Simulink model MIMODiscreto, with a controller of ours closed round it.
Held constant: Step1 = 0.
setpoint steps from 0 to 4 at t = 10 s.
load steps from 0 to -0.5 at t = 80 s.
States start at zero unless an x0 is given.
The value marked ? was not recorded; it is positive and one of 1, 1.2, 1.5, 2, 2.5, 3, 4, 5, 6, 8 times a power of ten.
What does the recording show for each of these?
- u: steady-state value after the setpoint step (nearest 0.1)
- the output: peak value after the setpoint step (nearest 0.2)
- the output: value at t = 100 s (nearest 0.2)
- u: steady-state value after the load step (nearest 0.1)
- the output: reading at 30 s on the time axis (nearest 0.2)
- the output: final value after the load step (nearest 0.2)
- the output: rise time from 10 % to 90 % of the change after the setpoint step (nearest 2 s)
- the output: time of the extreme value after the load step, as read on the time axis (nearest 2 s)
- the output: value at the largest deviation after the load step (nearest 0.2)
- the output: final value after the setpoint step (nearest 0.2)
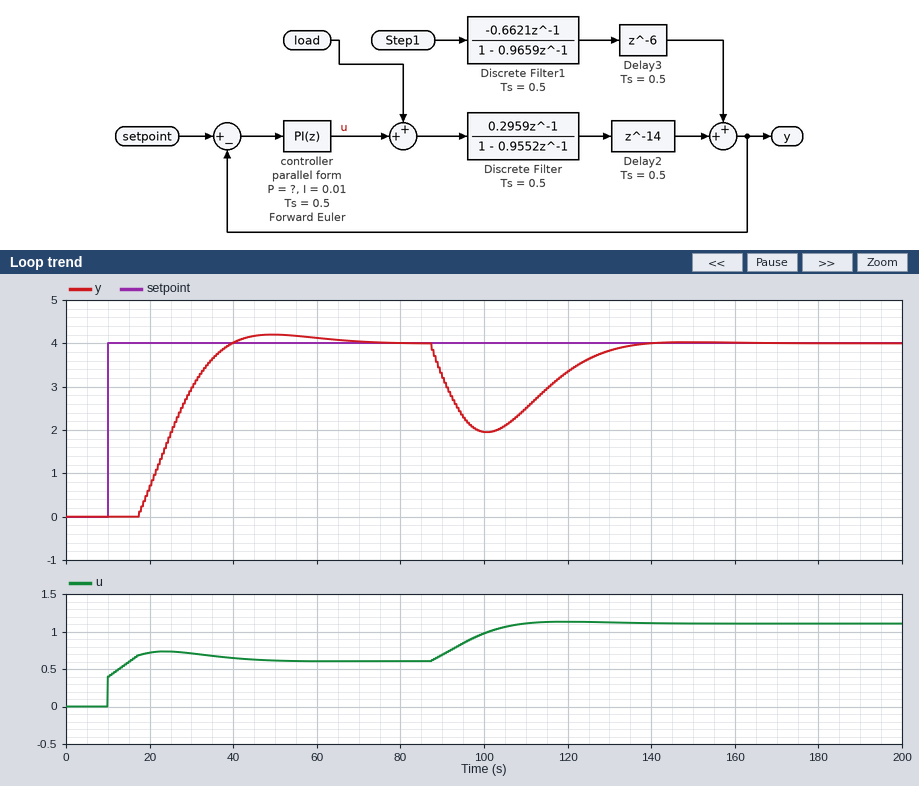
0.6
4.2
2.0
1.1
3.0
4.0
16 s
100 s
2.0
4.0
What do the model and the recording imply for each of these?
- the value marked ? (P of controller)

0.1
